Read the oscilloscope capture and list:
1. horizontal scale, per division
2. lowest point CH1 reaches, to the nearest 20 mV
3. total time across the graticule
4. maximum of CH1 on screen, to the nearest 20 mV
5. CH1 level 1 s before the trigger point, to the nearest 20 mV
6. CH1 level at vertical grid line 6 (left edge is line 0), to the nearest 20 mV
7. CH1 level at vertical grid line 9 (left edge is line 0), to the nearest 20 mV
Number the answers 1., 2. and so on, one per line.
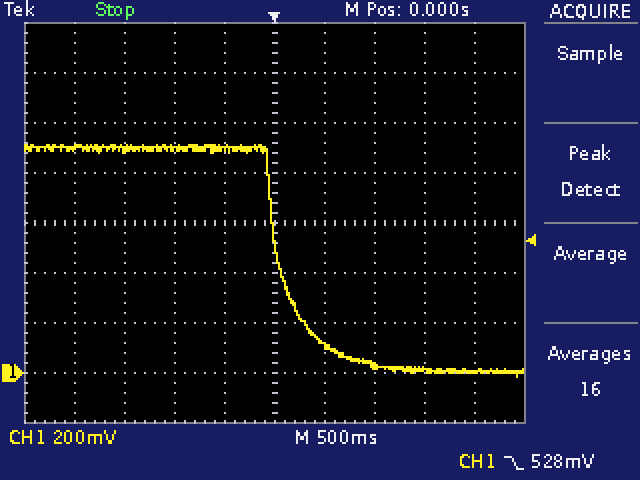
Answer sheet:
1. 500 ms
2. -20 mV
3. 5 s
4. 920 mV
5. 900 mV
6. 120 mV
7. 0 mV
